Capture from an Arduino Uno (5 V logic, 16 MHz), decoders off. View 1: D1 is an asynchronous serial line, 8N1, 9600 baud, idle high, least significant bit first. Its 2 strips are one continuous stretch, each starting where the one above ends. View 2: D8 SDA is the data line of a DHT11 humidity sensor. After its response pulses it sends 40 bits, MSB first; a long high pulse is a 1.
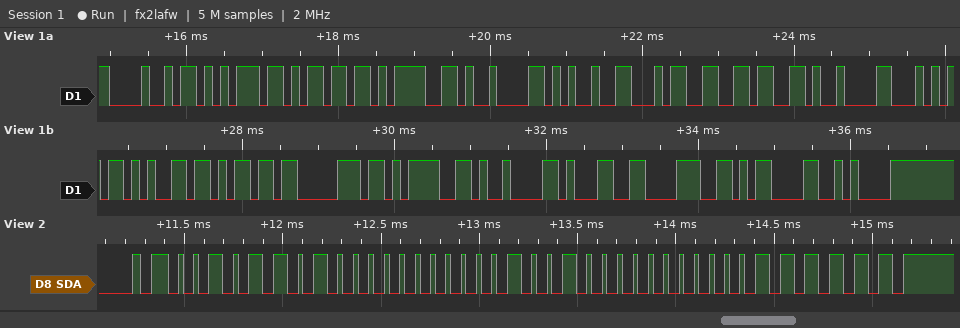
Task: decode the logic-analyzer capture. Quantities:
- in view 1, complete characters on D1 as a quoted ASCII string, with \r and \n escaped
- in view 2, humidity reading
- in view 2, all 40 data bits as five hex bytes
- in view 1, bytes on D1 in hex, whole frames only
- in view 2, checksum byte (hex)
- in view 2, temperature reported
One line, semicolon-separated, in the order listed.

"Hum=\t%46\tTemp=\t18\r\n"; 45 %; 2D 00 12 00 3F; 0x48 0x75 0x6D 0x3D 0x09 0x25 0x34 0x36 0x09 0x54 0x65 0x6D 0x70 0x3D 0x09 0x31 0x38 0x0D 0x0A; 0x3F; 18.0 °C
